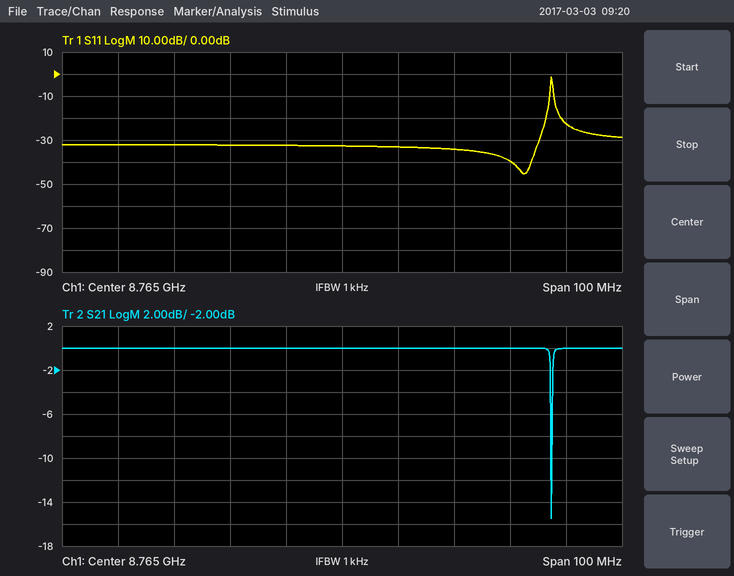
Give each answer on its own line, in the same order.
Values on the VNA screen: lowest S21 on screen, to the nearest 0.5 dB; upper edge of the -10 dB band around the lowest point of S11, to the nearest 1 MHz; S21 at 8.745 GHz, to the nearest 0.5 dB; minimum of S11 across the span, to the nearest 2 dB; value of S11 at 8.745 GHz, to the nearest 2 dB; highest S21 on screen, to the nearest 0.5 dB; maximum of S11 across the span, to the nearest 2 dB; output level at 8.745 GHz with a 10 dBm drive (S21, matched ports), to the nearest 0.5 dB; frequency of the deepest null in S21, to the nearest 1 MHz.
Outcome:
-15.5 dB
8.802 GHz
0.0 dB
-46 dB
-32 dB
0.0 dB
-2 dB
10.0 dBm
8.802 GHz
